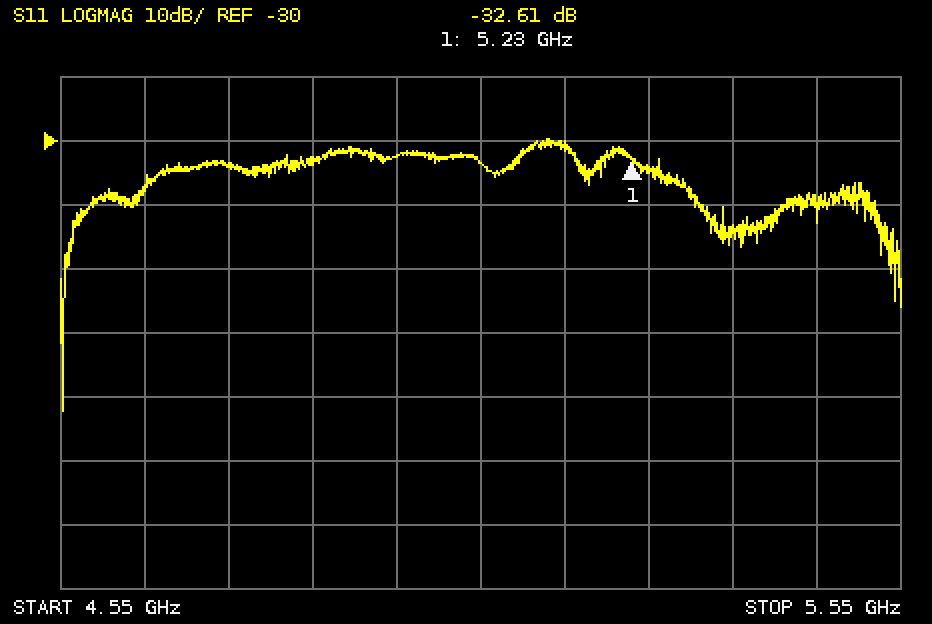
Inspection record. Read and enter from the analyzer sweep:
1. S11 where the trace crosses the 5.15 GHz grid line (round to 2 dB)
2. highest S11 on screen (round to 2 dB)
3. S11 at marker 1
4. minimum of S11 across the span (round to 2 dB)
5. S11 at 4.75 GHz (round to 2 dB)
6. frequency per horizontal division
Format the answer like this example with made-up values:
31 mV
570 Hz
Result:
-30 dB
-30 dB
-32.61 dB
-72 dB
-34 dB
100 MHz
